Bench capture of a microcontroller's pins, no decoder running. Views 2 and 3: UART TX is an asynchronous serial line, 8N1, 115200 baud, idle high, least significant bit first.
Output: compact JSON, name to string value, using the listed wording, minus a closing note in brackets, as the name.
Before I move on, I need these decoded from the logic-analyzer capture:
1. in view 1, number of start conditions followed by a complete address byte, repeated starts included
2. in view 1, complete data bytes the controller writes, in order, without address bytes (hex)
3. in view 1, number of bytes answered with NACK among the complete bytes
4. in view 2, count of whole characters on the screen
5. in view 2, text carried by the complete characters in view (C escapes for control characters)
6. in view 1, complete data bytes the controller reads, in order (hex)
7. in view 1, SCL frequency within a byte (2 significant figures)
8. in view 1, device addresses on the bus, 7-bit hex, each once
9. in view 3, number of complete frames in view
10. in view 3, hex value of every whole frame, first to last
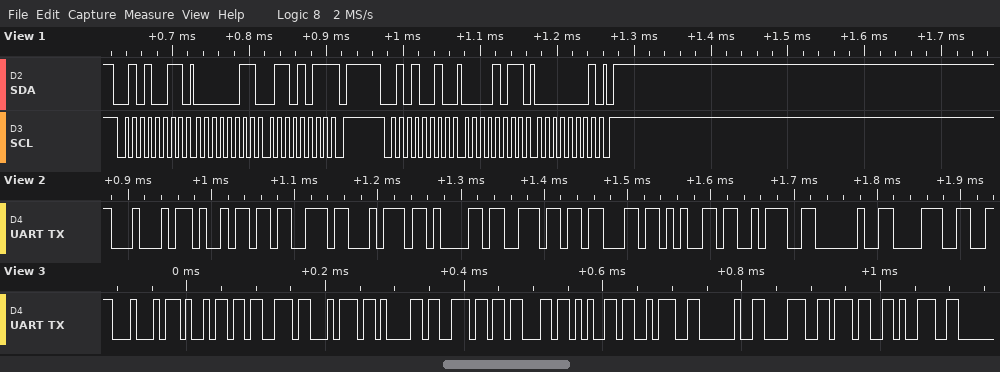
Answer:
{"in view 1, number of start conditions followed by a complete address byte, repeated starts included": "2", "in view 1, complete data bytes the controller writes, in order, without address bytes": "0B 01", "in view 1, number of bytes answered with NACK among the complete bytes": "1", "in view 2, count of whole characters on the screen": "11", "in view 2, text carried by the complete characters in view": "\"Distance: 8\"", "in view 1, complete data bytes the controller reads, in order": "03 6B", "in view 1, SCL frequency within a byte": "100 kHz", "in view 1, device addresses on the bus, 7-bit hex, each once": "0x29", "in view 3, number of complete frames in view": "13", "in view 3, hex value of every whole frame, first to last": "44 69 73 74 61 6E 63 65 3A 20 38 37 39"}
